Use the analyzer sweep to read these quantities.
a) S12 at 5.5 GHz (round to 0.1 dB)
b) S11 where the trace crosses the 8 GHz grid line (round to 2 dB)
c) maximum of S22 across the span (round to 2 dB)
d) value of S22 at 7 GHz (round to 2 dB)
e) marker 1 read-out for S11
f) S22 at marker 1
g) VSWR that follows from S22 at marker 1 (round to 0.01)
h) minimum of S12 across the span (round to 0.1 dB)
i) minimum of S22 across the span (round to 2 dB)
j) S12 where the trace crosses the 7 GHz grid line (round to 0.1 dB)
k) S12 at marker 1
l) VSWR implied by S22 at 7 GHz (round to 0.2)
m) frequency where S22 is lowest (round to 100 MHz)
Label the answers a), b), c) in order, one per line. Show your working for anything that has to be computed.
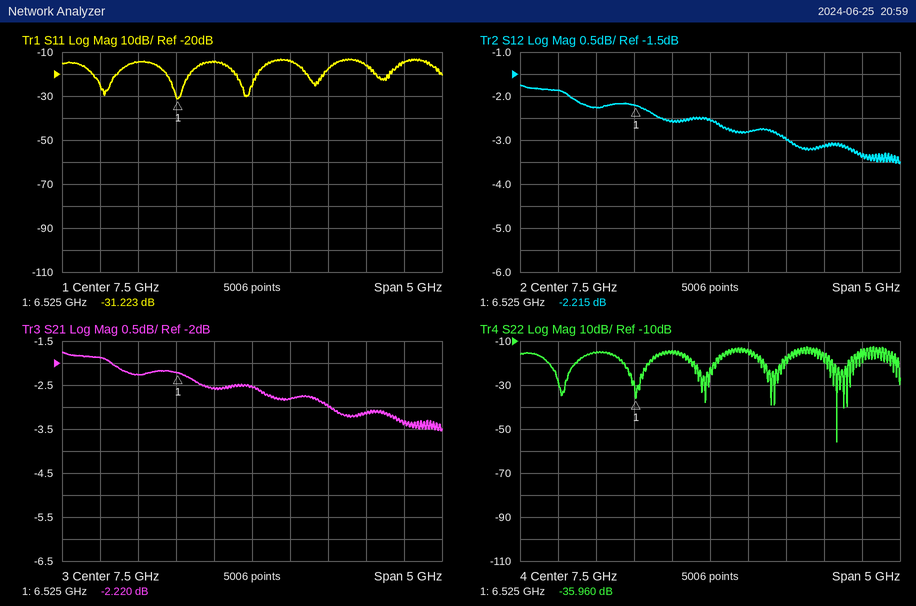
a) -1.9 dB
b) -14 dB
c) -12 dB
d) -14 dB
e) -31.223 dB
f) -35.960 dB
g) (1 + 0.0159)/(1 − 0.0159) ≈ 1.03
h) -3.5 dB
i) -56 dB
j) -2.6 dB
k) -2.215 dB
l) |Γ| = 10^(-14/20) = 0.1995; VSWR = (1 + 0.1995)/(1 − 0.1995) ≈ 1.50, so 1.4 to the nearest 0.2
m) 9.2 GHz
